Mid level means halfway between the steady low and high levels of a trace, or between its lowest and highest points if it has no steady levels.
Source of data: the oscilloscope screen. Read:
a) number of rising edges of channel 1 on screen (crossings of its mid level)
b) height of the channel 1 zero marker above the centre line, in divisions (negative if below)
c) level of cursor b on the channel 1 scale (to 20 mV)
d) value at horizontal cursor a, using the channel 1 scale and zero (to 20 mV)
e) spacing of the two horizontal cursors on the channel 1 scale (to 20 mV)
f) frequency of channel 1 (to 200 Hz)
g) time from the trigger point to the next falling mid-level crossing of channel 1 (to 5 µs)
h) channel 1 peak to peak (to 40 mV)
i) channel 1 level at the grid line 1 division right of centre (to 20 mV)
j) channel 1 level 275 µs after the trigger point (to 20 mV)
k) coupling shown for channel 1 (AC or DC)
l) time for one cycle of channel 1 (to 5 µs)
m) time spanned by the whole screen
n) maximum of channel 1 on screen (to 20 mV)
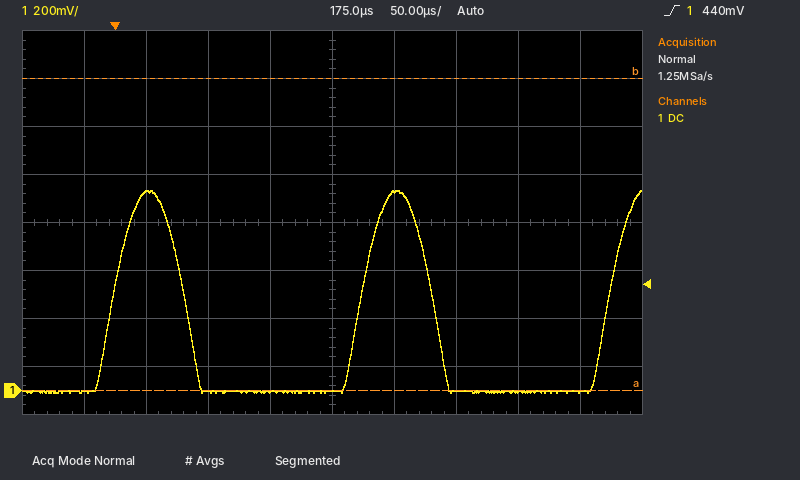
3
-3.5 div
1.30 V
0 mV
1.30 V
5.0 kHz
55 µs
840 mV
820 mV
0 mV
DC
200 µs
500 µs
840 mV
